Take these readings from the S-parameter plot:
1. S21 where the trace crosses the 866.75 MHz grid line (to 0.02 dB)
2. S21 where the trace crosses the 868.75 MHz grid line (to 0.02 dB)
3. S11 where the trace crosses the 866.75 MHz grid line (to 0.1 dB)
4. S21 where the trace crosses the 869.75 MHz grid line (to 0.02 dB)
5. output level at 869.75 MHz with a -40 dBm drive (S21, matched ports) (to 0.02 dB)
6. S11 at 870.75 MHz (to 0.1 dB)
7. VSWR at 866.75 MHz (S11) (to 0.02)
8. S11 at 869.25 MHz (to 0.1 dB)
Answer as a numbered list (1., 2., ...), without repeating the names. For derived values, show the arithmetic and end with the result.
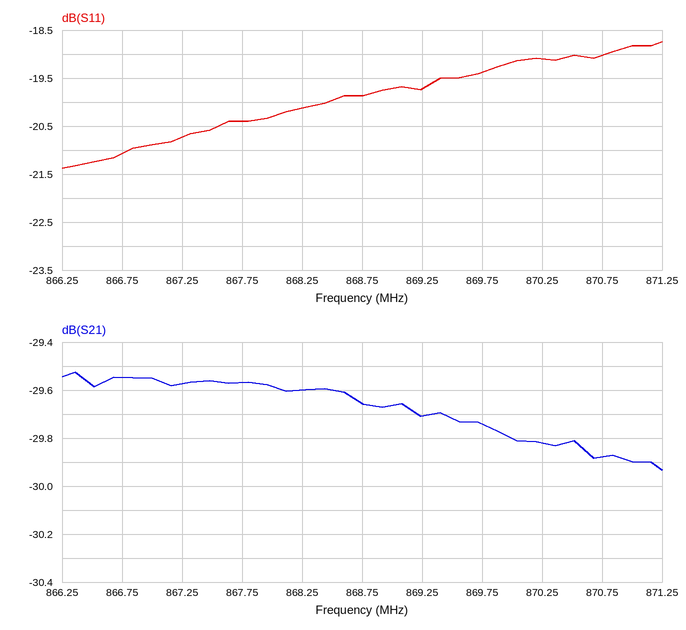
1. -29.54 dB
2. -29.66 dB
3. -21.1 dB
4. -29.74 dB
5. -40 dBm + (-29.74 dB) = -69.74 dBm
6. -19.0 dB
7. |Γ| = 10^(-21.1/20) = 0.0881; VSWR = (1 + 0.0881)/(1 − 0.0881) ≈ 1.19, so 1.20 to the nearest 0.02
8. -19.7 dB
